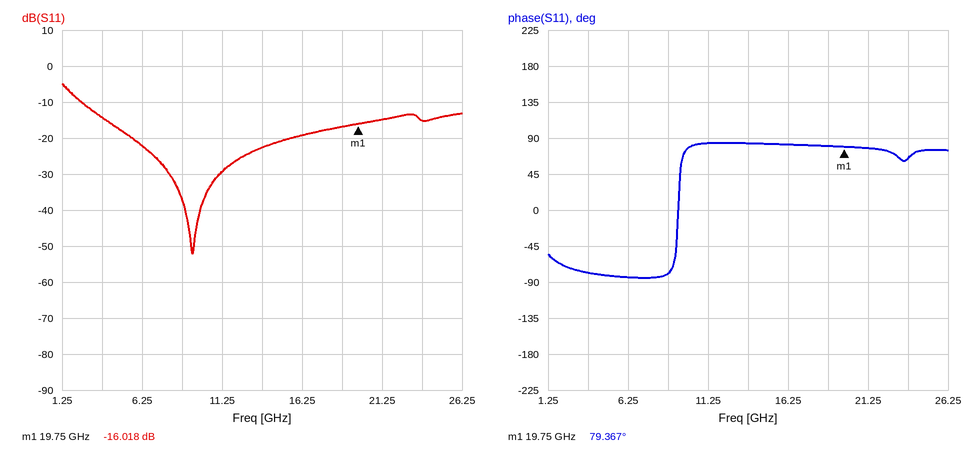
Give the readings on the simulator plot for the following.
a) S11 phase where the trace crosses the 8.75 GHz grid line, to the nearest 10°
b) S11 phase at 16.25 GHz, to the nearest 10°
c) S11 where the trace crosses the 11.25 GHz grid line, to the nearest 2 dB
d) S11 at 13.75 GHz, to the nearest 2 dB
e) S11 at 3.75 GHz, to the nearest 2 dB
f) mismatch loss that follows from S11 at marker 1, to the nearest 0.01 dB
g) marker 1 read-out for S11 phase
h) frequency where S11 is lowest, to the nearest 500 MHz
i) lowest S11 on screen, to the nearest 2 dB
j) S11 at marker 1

-80°
80°
-30 dB
-22 dB
-14 dB
0.11 dB
79.367°
9.5 GHz
-52 dB
-16.018 dB
